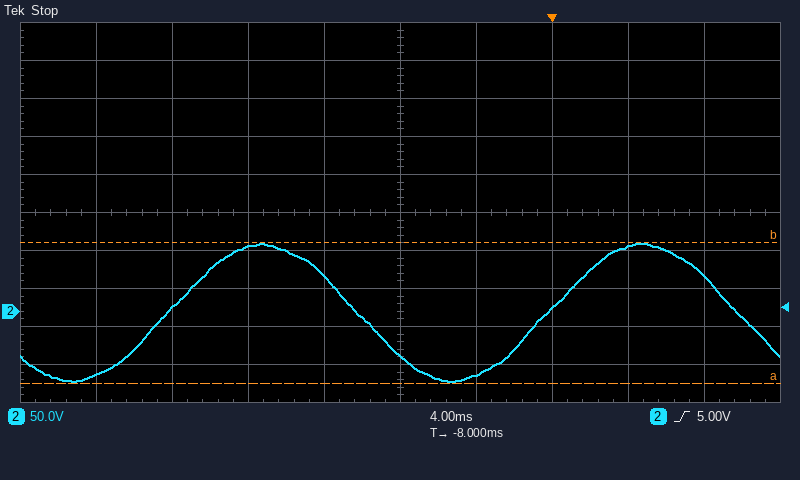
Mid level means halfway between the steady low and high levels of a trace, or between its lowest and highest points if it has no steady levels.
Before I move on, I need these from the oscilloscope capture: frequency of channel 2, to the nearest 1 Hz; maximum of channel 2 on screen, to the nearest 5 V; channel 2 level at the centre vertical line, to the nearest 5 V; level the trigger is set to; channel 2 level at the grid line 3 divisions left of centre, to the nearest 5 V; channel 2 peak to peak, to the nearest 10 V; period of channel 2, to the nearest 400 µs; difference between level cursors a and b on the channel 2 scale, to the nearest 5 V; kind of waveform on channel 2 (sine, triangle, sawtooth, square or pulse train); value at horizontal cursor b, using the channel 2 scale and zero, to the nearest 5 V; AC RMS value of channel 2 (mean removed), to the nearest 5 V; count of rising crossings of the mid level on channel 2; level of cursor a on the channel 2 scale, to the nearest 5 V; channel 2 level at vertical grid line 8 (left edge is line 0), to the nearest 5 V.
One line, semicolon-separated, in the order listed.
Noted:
50 Hz; 90 V; -60 V; 5.00 V; 5 V; 180 V; 20.0 ms; 185 V; sine; 90 V; 65 V; 2; -95 V; 85 V
